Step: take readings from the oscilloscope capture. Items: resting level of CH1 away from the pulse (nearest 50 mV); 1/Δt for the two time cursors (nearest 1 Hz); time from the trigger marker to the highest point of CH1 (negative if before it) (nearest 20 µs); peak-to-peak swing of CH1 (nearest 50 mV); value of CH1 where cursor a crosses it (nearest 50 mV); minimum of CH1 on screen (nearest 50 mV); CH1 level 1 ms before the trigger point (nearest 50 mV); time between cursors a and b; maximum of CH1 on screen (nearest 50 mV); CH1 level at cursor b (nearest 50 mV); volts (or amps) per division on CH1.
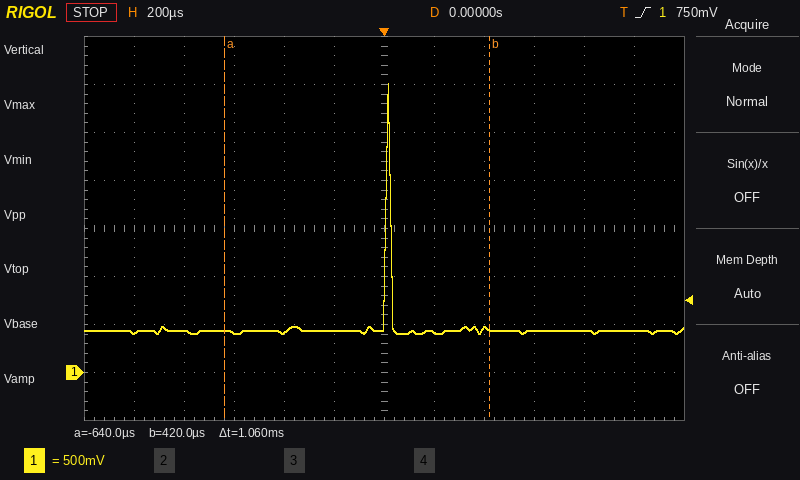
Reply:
450 mV
943 Hz
+20 µs
2.60 V
450 mV
400 mV
400 mV
1.06 ms
3.00 V
450 mV
500 mV
